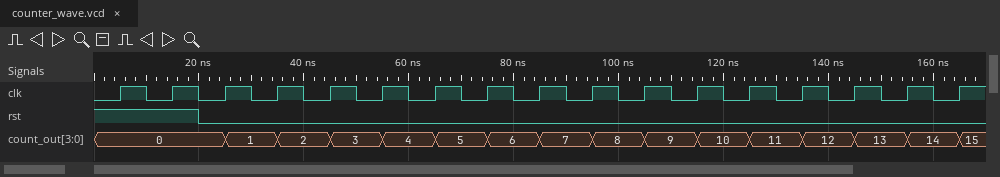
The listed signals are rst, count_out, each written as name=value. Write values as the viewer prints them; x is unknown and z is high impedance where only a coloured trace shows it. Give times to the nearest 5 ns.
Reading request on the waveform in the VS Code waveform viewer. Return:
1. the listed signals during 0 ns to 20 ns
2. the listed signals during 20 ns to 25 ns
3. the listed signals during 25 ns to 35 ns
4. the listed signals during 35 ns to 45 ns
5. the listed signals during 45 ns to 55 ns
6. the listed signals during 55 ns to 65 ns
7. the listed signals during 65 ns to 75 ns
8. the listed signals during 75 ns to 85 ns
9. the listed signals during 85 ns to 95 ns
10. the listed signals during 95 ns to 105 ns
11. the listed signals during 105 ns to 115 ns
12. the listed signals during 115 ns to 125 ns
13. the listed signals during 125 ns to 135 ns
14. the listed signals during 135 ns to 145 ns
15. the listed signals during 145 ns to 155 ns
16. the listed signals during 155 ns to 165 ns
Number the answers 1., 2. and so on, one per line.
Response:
1. rst=1, count_out=0
2. rst=0, count_out=0
3. rst=0, count_out=1
4. rst=0, count_out=2
5. rst=0, count_out=3
6. rst=0, count_out=4
7. rst=0, count_out=5
8. rst=0, count_out=6
9. rst=0, count_out=7
10. rst=0, count_out=8
11. rst=0, count_out=9
12. rst=0, count_out=10
13. rst=0, count_out=11
14. rst=0, count_out=12
15. rst=0, count_out=13
16. rst=0, count_out=14
